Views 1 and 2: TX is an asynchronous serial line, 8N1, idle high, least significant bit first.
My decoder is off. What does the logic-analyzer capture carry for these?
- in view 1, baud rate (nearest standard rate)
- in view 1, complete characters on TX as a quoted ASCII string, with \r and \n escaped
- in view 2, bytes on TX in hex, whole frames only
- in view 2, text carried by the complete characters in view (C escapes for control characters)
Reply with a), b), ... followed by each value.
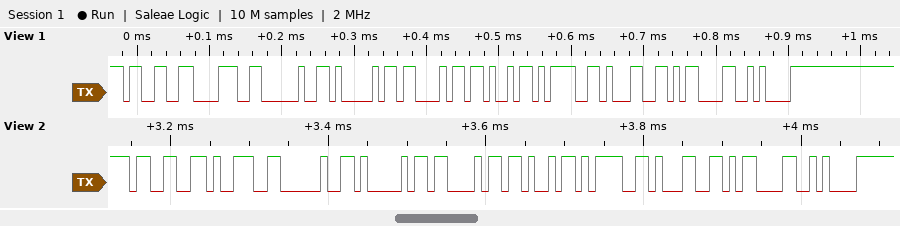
a) 115200 baud
b) "38 ACK=1\r\n"
c) 33 39 20 41 43 4B 3D 31 0D 0A
d) "39 ACK=1\r\n"
